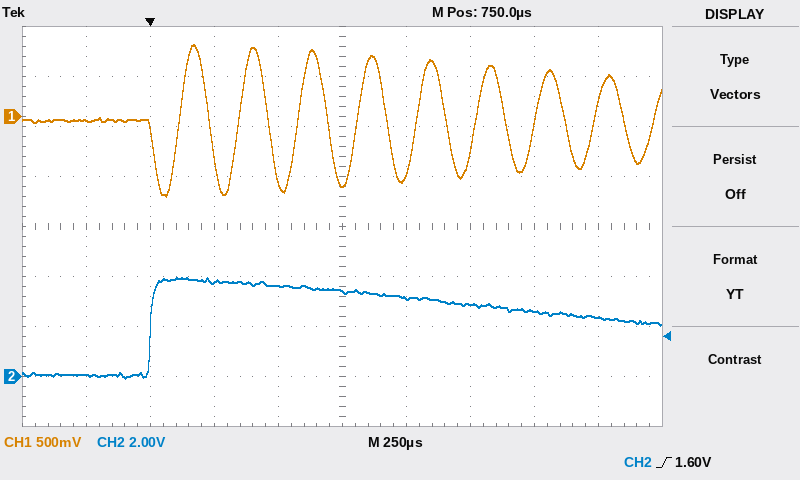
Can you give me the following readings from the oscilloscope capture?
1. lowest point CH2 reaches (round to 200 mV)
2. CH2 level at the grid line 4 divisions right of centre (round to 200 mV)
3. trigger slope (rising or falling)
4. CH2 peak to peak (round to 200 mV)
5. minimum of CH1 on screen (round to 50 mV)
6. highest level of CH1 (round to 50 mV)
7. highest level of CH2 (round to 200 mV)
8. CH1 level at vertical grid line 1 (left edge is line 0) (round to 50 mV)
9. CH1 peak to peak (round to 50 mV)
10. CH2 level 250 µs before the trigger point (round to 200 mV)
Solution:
0.0 V
2.4 V
rising
4.0 V
-800 mV
700 mV
4.0 V
-50 mV
1.50 V
0.0 V
